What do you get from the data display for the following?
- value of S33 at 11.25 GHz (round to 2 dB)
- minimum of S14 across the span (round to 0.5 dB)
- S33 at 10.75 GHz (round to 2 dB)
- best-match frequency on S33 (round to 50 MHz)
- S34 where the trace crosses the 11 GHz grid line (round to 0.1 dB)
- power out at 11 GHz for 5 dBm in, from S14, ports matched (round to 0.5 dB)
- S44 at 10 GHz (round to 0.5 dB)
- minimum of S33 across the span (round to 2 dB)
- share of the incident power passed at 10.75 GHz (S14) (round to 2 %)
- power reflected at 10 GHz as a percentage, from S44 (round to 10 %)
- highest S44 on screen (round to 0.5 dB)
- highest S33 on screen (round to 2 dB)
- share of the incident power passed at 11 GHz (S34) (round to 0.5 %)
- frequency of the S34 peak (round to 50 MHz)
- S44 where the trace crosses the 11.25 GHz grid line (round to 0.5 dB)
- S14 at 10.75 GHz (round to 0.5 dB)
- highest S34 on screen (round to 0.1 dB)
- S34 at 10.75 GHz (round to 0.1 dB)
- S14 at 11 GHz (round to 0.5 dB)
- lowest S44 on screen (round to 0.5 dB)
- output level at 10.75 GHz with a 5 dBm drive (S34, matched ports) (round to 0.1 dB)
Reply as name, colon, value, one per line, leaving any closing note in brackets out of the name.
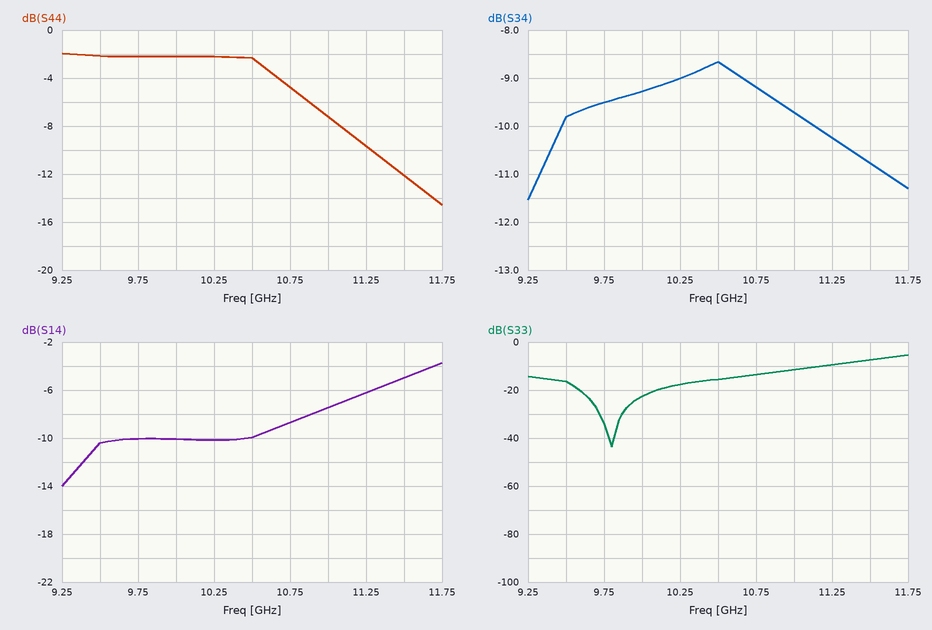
value of S33 at 11.25 GHz: -10 dB
minimum of S14 across the span: -14.0 dB
S33 at 10.75 GHz: -14 dB
best-match frequency on S33: 9.80 GHz
S34 where the trace crosses the 11 GHz grid line: -9.7 dB
power out at 11 GHz for 5 dBm in, from S14, ports matched: -2.5 dBm
S44 at 10 GHz: -2.0 dB
minimum of S33 across the span: -44 dB
share of the incident power passed at 10.75 GHz (S14): 14 %
power reflected at 10 GHz as a percentage, from S44: 60 %
highest S44 on screen: -2.0 dB
highest S33 on screen: -6 dB
share of the incident power passed at 11 GHz (S34): 10.5 %
frequency of the S34 peak: 10.50 GHz
S44 where the trace crosses the 11.25 GHz grid line: -9.5 dB
S14 at 10.75 GHz: -8.5 dB
highest S34 on screen: -8.7 dB
S34 at 10.75 GHz: -9.2 dB
S14 at 11 GHz: -7.5 dB
lowest S44 on screen: -14.5 dB
output level at 10.75 GHz with a 5 dBm drive (S34, matched ports): -4.2 dBm
